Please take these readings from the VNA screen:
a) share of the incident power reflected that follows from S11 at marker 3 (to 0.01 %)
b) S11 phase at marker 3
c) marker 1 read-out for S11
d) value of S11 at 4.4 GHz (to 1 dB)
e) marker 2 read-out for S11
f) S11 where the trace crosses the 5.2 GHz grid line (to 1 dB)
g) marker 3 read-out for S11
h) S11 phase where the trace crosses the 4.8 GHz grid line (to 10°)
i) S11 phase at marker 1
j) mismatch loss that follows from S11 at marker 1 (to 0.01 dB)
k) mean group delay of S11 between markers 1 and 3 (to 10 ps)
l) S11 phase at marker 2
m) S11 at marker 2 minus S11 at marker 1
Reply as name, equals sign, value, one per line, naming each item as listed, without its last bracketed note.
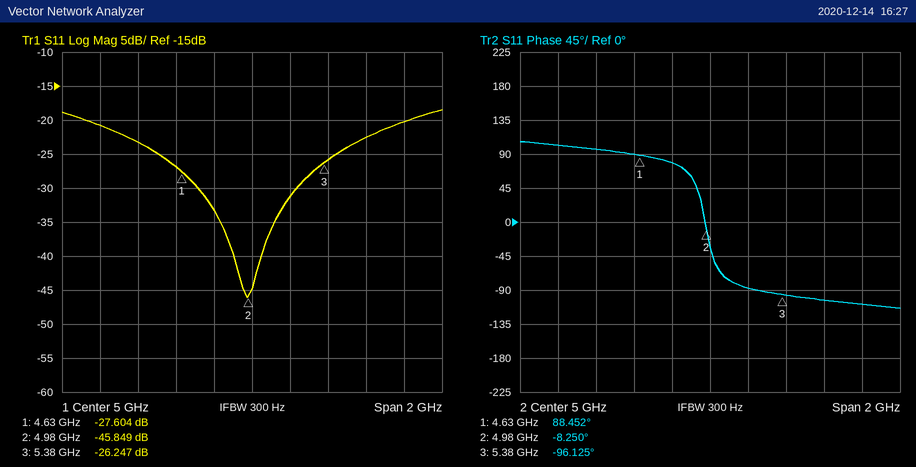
share of the incident power reflected that follows from S11 at marker 3 = 0.24 %
S11 phase at marker 3 = -96.125°
marker 1 read-out for S11 = -27.604 dB
value of S11 at 4.4 GHz = -23 dB
marker 2 read-out for S11 = -45.849 dB
S11 where the trace crosses the 5.2 GHz grid line = -31 dB
marker 3 read-out for S11 = -26.247 dB
S11 phase where the trace crosses the 4.8 GHz grid line = 80°
S11 phase at marker 1 = 88.452°
mismatch loss that follows from S11 at marker 1 = 0.01 dB
mean group delay of S11 between markers 1 and 3 = 680 ps
S11 phase at marker 2 = -8.250°
S11 at marker 2 minus S11 at marker 1 = -18.245 dB
